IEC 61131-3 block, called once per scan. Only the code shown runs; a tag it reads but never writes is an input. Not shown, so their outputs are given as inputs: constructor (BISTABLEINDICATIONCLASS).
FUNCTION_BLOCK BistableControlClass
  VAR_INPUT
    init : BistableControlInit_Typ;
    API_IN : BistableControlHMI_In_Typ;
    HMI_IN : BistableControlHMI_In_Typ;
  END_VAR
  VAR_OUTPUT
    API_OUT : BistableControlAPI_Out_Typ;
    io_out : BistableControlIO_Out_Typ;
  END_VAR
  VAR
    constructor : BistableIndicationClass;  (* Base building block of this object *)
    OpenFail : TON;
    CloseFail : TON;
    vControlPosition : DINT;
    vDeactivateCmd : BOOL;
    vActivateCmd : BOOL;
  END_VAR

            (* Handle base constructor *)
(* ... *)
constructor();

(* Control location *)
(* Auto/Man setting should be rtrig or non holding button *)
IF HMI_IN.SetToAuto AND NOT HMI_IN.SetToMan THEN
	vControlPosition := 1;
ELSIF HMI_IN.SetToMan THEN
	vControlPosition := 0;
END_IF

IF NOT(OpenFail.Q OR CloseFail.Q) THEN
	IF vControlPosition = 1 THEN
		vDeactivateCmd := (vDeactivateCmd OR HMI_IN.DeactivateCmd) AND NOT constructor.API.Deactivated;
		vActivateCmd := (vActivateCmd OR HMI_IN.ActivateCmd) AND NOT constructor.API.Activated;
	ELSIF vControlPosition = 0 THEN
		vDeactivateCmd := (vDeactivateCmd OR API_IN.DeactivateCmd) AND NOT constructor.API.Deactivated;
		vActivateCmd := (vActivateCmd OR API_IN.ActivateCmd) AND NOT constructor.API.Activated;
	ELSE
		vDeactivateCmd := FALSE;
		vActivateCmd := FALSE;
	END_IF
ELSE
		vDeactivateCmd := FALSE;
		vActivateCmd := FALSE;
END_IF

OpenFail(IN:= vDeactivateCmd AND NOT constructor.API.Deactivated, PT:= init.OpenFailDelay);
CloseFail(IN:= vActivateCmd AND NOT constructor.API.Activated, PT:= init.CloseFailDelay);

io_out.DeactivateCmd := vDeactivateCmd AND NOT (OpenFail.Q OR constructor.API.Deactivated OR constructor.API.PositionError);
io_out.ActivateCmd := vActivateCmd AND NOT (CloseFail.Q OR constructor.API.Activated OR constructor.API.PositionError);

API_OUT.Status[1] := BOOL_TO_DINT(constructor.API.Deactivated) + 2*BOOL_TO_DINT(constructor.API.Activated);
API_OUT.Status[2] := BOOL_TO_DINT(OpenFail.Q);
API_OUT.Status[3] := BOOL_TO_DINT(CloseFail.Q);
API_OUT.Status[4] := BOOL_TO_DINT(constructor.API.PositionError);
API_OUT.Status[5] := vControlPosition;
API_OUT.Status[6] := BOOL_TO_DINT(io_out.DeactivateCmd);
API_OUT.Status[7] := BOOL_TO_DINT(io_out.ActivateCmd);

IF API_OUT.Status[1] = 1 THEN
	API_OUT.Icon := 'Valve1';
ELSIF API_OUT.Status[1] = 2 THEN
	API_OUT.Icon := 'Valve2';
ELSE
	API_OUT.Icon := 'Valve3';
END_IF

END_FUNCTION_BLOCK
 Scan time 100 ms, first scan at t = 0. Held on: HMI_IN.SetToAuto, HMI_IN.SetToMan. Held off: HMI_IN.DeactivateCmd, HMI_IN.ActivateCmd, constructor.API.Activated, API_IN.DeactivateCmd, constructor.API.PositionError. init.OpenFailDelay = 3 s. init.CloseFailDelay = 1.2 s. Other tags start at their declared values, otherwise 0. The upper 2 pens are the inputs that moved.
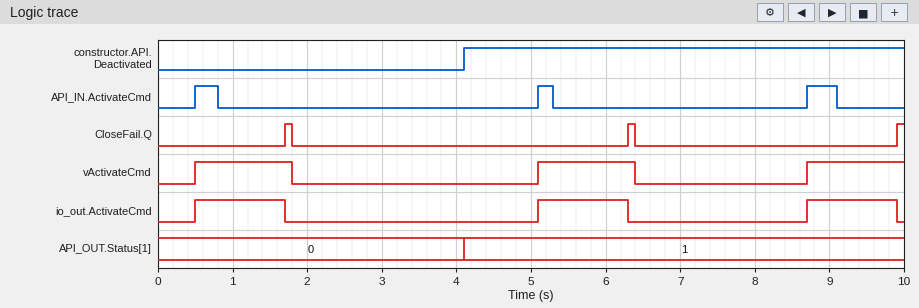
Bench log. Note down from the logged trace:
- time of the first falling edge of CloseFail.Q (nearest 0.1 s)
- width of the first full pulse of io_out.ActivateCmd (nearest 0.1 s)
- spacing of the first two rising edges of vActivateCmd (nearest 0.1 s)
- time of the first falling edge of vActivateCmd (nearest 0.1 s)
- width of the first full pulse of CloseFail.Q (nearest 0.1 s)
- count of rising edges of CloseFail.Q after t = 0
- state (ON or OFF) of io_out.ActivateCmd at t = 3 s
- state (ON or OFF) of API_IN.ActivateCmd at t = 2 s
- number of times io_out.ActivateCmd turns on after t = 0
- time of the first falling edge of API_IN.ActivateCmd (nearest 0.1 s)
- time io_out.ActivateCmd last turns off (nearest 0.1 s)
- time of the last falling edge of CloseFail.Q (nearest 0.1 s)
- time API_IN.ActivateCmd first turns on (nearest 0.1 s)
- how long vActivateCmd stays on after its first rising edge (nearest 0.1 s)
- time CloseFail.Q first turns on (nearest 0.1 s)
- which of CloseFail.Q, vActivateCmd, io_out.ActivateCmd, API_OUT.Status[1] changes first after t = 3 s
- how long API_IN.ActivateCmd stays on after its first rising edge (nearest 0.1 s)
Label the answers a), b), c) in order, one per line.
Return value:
a) 1.8 s
b) 1.2 s
c) 4.6 s
d) 1.8 s
e) 0.1 s
f) 3
g) OFF
h) OFF
i) 3
j) 0.8 s
k) 9.9 s
l) 6.4 s
m) 0.5 s
n) 1.3 s
o) 1.7 s
p) API_OUT.Status[1]
q) 0.3 s
